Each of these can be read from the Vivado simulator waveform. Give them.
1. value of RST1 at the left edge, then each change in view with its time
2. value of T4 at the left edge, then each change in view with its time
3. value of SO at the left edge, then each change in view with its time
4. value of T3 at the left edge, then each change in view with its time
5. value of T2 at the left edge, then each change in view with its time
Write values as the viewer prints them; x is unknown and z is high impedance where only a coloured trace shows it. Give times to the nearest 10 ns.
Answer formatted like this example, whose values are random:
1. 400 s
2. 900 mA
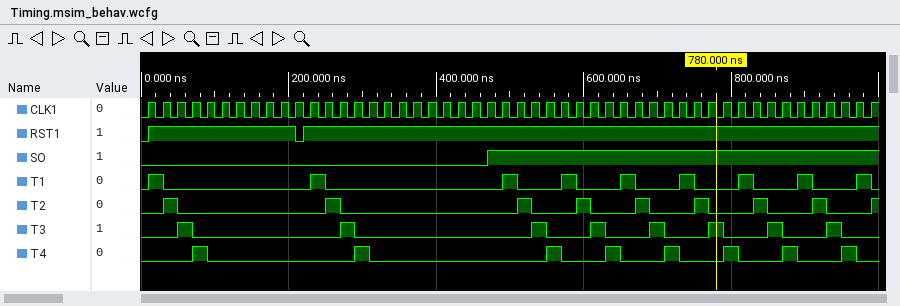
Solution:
1. 0, 1 at 10 ns, 0 at 210 ns, 1 at 220 ns
2. 0, 1 at 70 ns, 0 at 90 ns, 1 at 290 ns, 0 at 310 ns, 1 at 550 ns, 0 at 570 ns, 1 at 630 ns, 0 at 650 ns, 1 at 710 ns, 0 at 730 ns, 1 at 790 ns, 0 at 810 ns, 1 at 870 ns, 0 at 890 ns, 1 at 950 ns, 0 at 970 ns
3. 0, 1 at 470 ns
4. 0, 1 at 50 ns, 0 at 70 ns, 1 at 270 ns, 0 at 290 ns, 1 at 530 ns, 0 at 550 ns, 1 at 610 ns, 0 at 630 ns, 1 at 690 ns, 0 at 710 ns, 1 at 770 ns, 0 at 790 ns, 1 at 850 ns, 0 at 870 ns, 1 at 930 ns, 0 at 950 ns
5. 0, 1 at 30 ns, 0 at 50 ns, 1 at 250 ns, 0 at 270 ns, 1 at 510 ns, 0 at 530 ns, 1 at 590 ns, 0 at 610 ns, 1 at 670 ns, 0 at 690 ns, 1 at 750 ns, 0 at 770 ns, 1 at 830 ns, 0 at 850 ns, 1 at 910 ns, 0 at 930 ns, 1 at 990 ns
